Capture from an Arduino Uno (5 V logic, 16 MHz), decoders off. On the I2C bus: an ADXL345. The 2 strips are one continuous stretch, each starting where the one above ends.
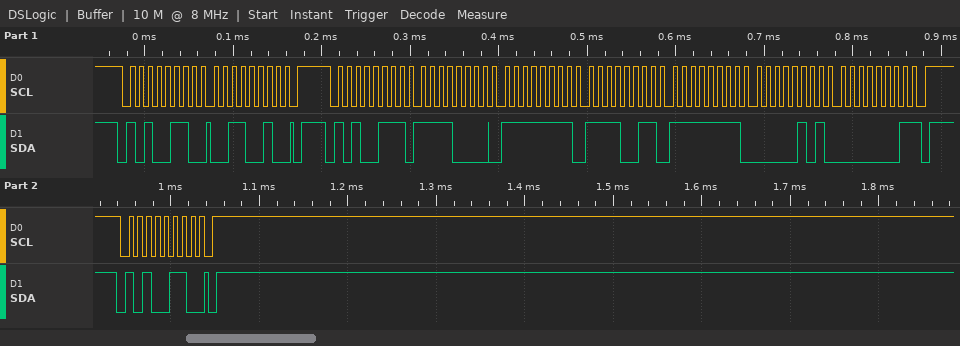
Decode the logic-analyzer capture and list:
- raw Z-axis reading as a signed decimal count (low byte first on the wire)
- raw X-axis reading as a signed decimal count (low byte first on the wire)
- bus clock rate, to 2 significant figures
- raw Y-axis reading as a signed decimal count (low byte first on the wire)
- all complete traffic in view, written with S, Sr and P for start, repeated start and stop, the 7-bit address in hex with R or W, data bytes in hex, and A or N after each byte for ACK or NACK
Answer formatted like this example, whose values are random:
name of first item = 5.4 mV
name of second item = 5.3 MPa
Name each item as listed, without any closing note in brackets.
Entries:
raw Z-axis reading as a signed decimal count = 261
raw X-axis reading as a signed decimal count = -16
bus clock rate, to 2 significant figures = 100 kHz
raw Y-axis reading as a signed decimal count = -13
all complete traffic in view, written with S, Sr and P for start, repeated start and stop, the 7-bit address in hex with R or W, data bytes in hex, and A or N after each byte for ACK or NACK = S 53W A 32 A P S 53R A F0 A FF A F3 A FF A 05 A 01 N P S 53W A P
